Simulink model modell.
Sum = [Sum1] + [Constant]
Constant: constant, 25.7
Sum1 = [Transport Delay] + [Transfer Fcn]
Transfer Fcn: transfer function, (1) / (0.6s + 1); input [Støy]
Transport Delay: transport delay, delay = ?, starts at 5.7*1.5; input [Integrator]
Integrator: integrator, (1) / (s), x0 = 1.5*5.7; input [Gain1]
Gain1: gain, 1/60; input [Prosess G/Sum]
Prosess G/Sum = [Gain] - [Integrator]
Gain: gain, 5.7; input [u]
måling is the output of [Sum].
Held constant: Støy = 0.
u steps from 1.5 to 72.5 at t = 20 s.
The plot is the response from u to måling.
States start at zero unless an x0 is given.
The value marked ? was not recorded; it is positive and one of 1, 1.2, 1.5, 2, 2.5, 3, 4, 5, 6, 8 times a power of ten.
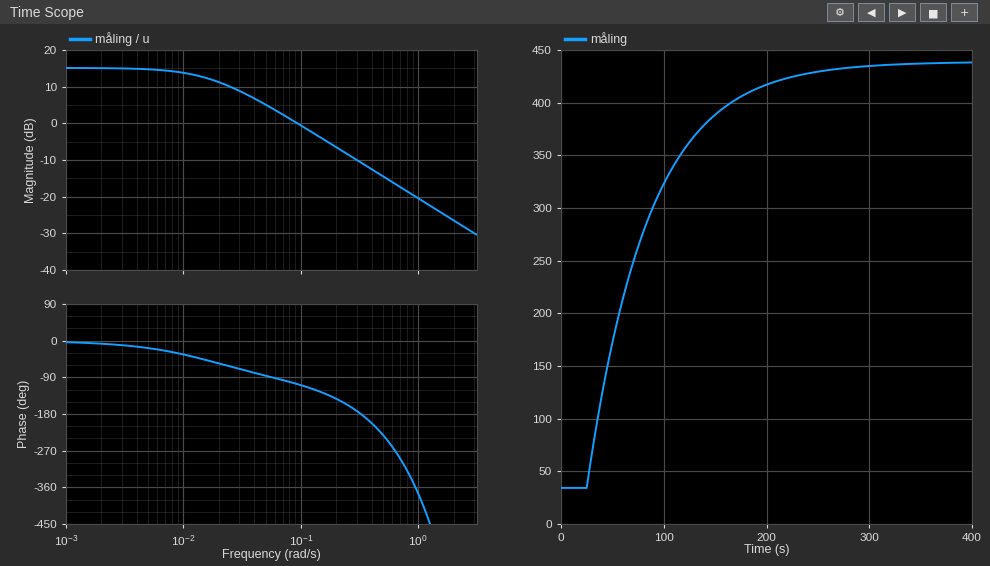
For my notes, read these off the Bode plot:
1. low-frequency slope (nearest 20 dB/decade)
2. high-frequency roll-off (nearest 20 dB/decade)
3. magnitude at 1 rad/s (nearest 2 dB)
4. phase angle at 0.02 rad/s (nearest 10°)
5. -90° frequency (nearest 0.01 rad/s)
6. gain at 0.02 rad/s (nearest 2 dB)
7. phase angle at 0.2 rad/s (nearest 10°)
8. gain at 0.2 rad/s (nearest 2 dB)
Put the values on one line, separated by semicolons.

0 dB/decade; -20 dB/decade; -20 dB; -60°; 0.06 rad/s; 12 dB; -140°; -6 dB
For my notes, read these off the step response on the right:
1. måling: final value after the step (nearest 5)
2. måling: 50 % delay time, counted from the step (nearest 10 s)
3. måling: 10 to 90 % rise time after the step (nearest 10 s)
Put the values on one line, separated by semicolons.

440; 50 s; 130 s
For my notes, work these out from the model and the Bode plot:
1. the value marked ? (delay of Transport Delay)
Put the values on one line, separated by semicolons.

5
